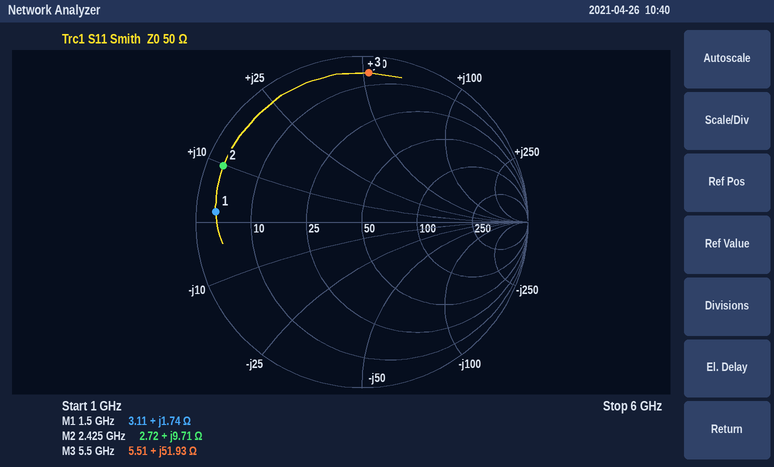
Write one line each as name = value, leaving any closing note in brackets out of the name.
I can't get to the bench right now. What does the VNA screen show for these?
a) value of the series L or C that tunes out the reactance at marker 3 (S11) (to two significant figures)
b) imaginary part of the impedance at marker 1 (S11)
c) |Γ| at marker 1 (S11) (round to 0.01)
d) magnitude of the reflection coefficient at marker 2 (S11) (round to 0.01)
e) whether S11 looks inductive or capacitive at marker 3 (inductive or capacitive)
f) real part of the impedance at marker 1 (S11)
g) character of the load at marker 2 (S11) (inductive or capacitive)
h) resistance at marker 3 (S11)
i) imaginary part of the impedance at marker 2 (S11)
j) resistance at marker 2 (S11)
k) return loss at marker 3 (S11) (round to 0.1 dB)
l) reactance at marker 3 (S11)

value of the series L or C that tunes out the reactance at marker 3 (S11) = 560 fF
imaginary part of the impedance at marker 1 = +1.74 Ω
|Γ| at marker 1 (S11) = 0.88
magnitude of the reflection coefficient at marker 2 (S11) = 0.90
whether S11 looks inductive or capacitive at marker 3 = inductive
real part of the impedance at marker 1 = 3.11 Ω
character of the load at marker 2 (S11) = inductive
resistance at marker 3 = 5.51 Ω
imaginary part of the impedance at marker 2 = +9.71 Ω
resistance at marker 2 = 2.72 Ω
return loss at marker 3 (S11) = 0.9 dB
reactance at marker 3 = +51.93 Ω
